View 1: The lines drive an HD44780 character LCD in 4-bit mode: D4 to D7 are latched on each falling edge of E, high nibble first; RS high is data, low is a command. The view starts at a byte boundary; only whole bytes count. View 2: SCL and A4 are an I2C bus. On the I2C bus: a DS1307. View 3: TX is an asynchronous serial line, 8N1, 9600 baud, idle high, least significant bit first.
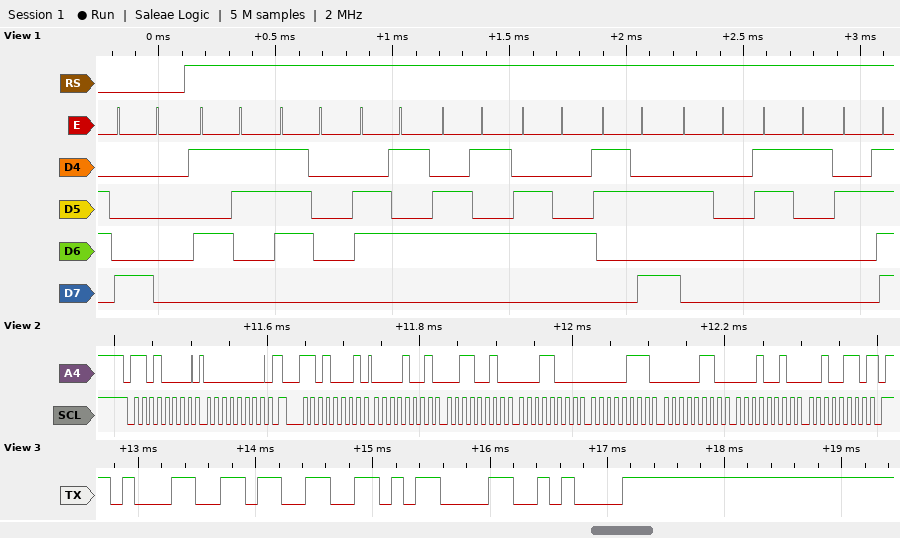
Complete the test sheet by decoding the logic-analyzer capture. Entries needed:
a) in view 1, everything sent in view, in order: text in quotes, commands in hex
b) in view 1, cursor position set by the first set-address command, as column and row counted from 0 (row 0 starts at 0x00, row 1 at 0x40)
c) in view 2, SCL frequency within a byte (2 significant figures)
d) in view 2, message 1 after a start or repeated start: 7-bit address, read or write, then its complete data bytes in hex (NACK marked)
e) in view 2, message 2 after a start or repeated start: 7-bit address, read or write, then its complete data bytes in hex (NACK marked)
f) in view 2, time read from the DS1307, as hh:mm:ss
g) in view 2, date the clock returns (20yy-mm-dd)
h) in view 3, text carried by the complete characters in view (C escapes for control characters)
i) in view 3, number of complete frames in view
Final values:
0x80 "Speed: 1/"
column 0, row 0
100 kHz
0x68 write: 00
0x68 read: 09 32 18 07 06 12 26 NACK
18:32:09
2026-12-06
"13\r\n"
4
